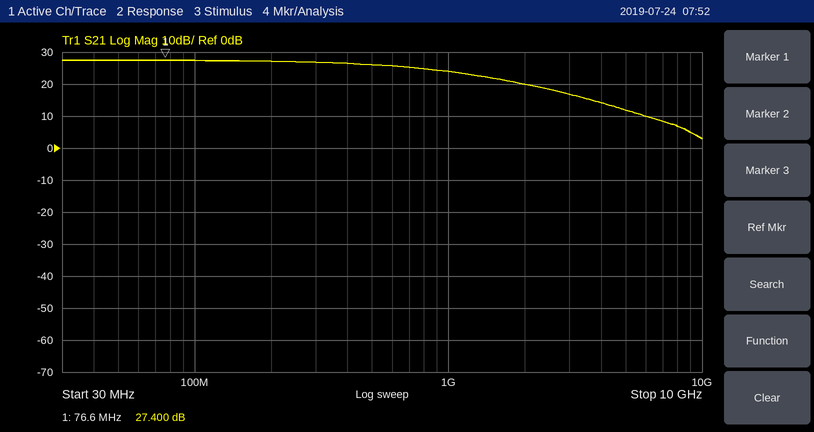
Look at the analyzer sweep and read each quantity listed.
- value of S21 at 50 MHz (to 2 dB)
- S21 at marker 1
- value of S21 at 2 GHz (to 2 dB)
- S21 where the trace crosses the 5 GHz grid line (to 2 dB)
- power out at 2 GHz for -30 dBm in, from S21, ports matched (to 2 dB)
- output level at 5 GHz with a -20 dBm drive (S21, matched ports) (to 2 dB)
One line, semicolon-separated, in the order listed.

28 dB; 27.400 dB; 20 dB; 12 dB; -10 dBm; -8 dBm
